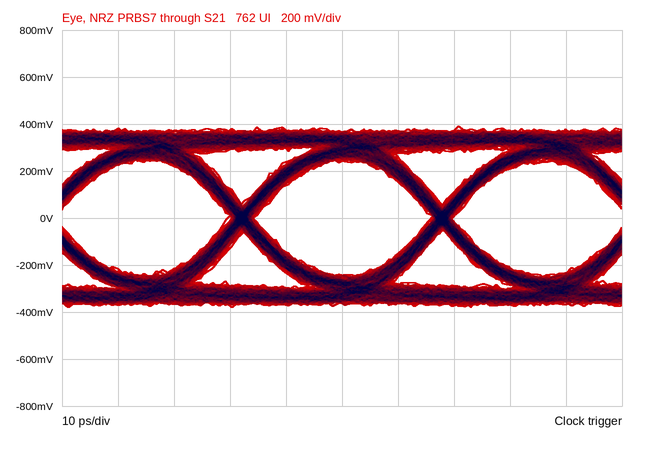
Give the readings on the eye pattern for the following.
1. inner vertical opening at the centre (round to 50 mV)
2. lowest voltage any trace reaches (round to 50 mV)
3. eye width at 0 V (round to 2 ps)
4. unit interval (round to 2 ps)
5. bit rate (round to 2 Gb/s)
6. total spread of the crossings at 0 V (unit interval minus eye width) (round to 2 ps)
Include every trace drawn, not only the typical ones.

500 mV
-400 mV
32 ps
36 ps
28 Gb/s
4 ps
